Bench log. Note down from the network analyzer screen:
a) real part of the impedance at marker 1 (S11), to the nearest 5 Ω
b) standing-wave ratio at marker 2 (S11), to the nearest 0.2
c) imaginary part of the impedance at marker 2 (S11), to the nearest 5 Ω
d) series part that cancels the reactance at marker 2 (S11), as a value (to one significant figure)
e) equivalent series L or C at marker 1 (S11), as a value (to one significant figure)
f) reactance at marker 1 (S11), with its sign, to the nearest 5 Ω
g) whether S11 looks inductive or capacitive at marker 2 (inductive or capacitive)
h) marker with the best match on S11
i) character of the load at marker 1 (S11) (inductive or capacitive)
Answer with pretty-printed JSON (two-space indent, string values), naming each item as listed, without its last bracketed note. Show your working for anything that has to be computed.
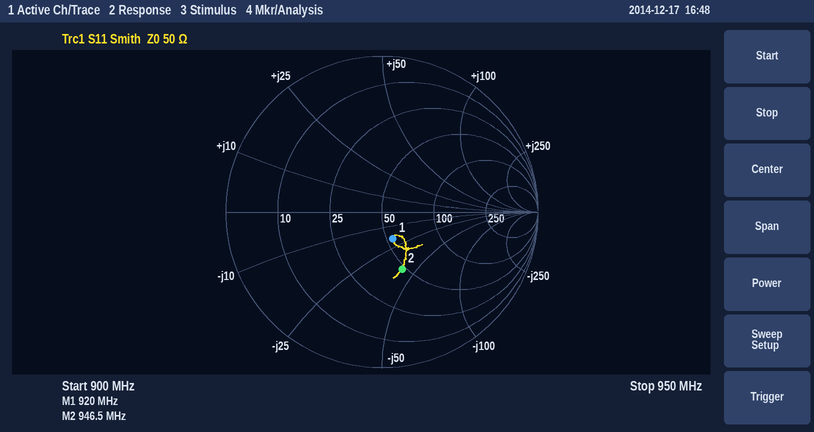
{
  "real part of the impedance at marker 1 (S11), to the nearest 5 Ω": "55 Ω",
  "standing-wave ratio at marker 2 (S11), to the nearest 0.2": "2.2",
  "imaginary part of the impedance at marker 2 (S11), to the nearest 5 Ω": "-40 Ω",
  "series part that cancels the reactance at marker 2 (S11), as a value": "L = 40 Ω/(2π × 946.5 MHz) ≈ 7 nH",
  "equivalent series L or C at marker 1 (S11), as a value": "C = 1/(2π × 920 MHz × 20 Ω) ≈ 9 pF",
  "reactance at marker 1 (S11), with its sign, to the nearest 5 Ω": "-20 Ω",
  "whether S11 looks inductive or capacitive at marker 2": "capacitive",
  "marker with the best match on S11": "marker 1",
  "character of the load at marker 1 (S11)": "capacitive"
}
